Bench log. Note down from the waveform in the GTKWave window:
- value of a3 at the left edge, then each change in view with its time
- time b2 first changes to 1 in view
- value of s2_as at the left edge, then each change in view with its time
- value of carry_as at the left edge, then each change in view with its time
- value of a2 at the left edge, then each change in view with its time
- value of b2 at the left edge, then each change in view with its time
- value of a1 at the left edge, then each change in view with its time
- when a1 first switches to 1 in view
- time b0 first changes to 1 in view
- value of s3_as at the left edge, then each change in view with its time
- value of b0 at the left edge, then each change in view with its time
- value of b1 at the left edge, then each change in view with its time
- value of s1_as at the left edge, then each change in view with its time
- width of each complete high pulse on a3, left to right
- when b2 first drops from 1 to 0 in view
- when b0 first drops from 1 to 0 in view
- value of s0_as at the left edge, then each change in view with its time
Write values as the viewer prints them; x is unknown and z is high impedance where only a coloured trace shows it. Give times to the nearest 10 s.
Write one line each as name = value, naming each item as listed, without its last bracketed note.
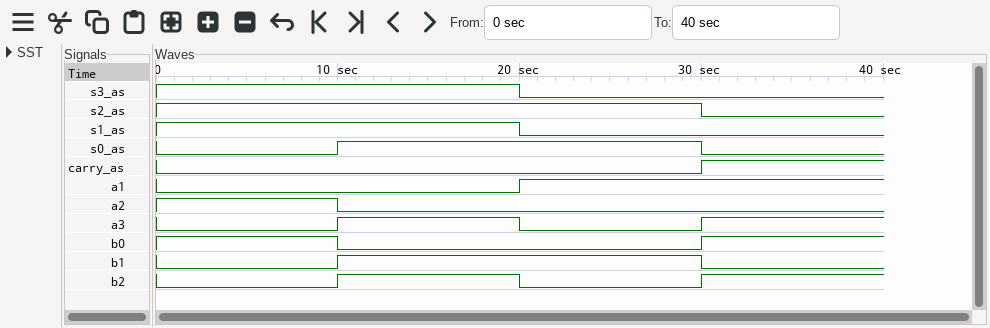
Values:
value of a3 at the left edge, then each change in view with its time = 0, 1 at 10 s, 0 at 20 s, 1 at 30 s
time b2 first changes to 1 in view = 10 s
value of s2_as at the left edge, then each change in view with its time = 1, 0 at 30 s
value of carry_as at the left edge, then each change in view with its time = 0, 1 at 30 s
value of a2 at the left edge, then each change in view with its time = 1, 0 at 10 s
value of b2 at the left edge, then each change in view with its time = 0, 1 at 10 s, 0 at 20 s, 1 at 30 s
value of a1 at the left edge, then each change in view with its time = 0, 1 at 20 s
when a1 first switches to 1 in view = 20 s
time b0 first changes to 1 in view = 30 s
value of s3_as at the left edge, then each change in view with its time = 1, 0 at 20 s
value of b0 at the left edge, then each change in view with its time = 1, 0 at 10 s, 1 at 30 s
value of b1 at the left edge, then each change in view with its time = 0, 1 at 10 s, 0 at 30 s
value of s1_as at the left edge, then each change in view with its time = 1, 0 at 20 s
width of each complete high pulse on a3, left to right = 10 s
when b2 first drops from 1 to 0 in view = 20 s
when b0 first drops from 1 to 0 in view = 10 s
value of s0_as at the left edge, then each change in view with its time = 0, 1 at 10 s, 0 at 30 s
